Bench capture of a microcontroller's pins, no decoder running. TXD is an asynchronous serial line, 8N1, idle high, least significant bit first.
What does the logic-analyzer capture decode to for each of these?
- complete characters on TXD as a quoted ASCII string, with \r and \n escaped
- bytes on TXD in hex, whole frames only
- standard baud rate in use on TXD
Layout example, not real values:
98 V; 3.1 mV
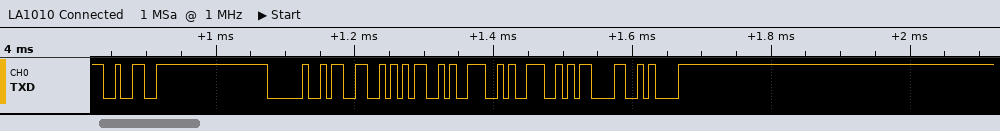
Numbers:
"2 3599\r\n"; 0x32 0x20 0x33 0x35 0x39 0x39 0x0D 0x0A; 115200 baud
